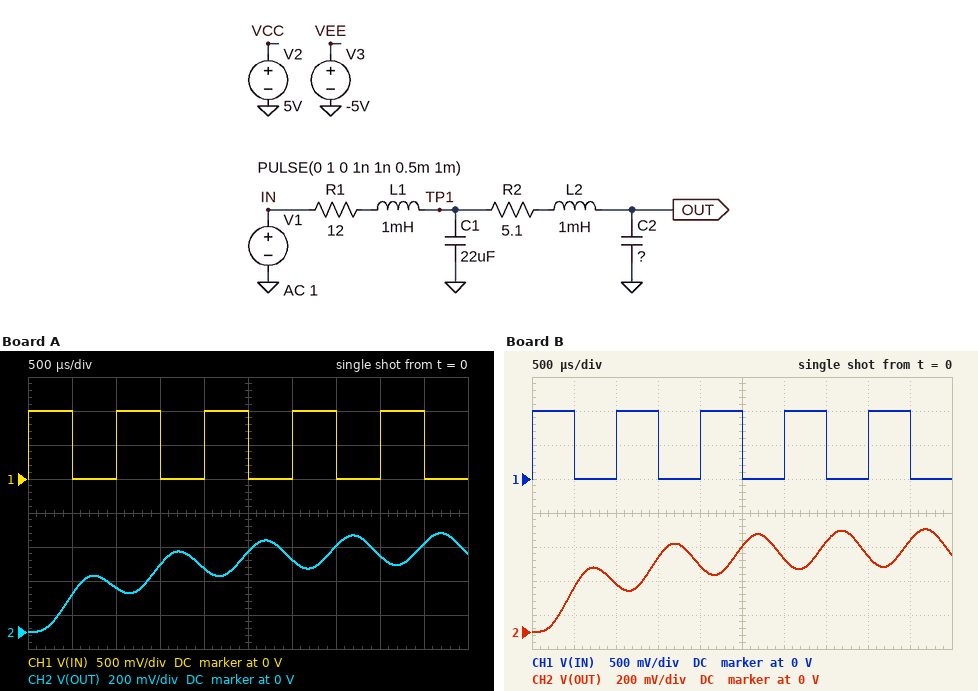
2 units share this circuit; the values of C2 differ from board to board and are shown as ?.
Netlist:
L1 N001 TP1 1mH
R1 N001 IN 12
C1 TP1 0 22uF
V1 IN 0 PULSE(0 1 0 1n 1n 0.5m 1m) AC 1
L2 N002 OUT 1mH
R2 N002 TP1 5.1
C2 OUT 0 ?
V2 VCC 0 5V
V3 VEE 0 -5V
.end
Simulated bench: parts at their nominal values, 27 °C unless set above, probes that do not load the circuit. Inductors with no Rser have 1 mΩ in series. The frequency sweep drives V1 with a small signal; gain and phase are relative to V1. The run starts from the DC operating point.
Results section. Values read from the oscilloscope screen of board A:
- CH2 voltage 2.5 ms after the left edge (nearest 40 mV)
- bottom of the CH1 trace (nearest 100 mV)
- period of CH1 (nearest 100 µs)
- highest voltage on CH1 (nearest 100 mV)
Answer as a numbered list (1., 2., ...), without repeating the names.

1. 480 mV
2. 0 V
3. 1.0 ms
4. 1.0 V
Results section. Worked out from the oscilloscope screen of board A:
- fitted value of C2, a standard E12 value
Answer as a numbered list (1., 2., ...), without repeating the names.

1. 68 µF
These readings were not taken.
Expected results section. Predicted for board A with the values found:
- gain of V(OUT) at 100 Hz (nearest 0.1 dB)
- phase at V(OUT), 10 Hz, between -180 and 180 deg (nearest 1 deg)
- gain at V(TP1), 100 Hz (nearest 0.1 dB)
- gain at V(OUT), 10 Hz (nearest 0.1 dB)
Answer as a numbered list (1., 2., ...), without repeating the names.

1. -2.1 dB
2. -5 deg
3. -2.1 dB
4. 0 dB
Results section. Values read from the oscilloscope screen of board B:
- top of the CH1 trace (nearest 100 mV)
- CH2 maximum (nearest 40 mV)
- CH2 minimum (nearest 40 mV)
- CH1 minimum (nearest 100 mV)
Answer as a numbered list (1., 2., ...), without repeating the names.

1. 1.0 V
2. 600 mV
3. 0 V
4. 0 V
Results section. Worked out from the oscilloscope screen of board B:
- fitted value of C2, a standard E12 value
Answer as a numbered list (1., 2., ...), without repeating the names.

1. 56 µF
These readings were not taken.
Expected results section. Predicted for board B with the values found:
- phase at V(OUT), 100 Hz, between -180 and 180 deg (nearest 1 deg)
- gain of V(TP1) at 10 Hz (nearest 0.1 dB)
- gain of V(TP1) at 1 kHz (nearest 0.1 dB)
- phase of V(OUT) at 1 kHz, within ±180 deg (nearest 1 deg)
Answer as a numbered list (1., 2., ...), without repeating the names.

1. -40 deg
2. 0 dB
3. -8.7 dB
4. -155 deg
